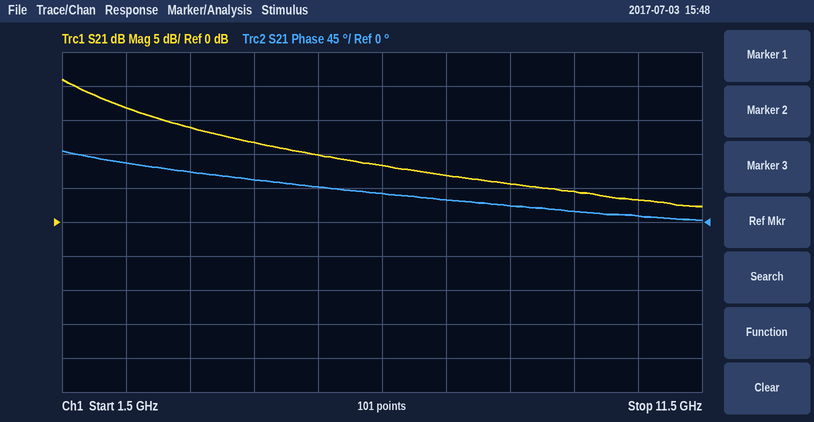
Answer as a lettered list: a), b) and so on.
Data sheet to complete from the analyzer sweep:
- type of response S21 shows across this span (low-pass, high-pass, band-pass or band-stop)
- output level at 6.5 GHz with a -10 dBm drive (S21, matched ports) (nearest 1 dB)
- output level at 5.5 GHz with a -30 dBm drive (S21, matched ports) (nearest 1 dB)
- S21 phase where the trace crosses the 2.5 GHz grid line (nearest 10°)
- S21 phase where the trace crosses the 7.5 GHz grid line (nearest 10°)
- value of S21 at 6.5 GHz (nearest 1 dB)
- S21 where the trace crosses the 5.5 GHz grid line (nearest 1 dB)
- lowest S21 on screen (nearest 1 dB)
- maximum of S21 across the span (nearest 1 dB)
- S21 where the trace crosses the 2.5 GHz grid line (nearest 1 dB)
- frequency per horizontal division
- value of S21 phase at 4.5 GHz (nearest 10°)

a) low-pass
b) -2 dBm
c) -20 dBm
d) 80°
e) 30°
f) 8 dB
g) 10 dB
h) 2 dB
i) 21 dB
j) 17 dB
k) 1 GHz
l) 60°
